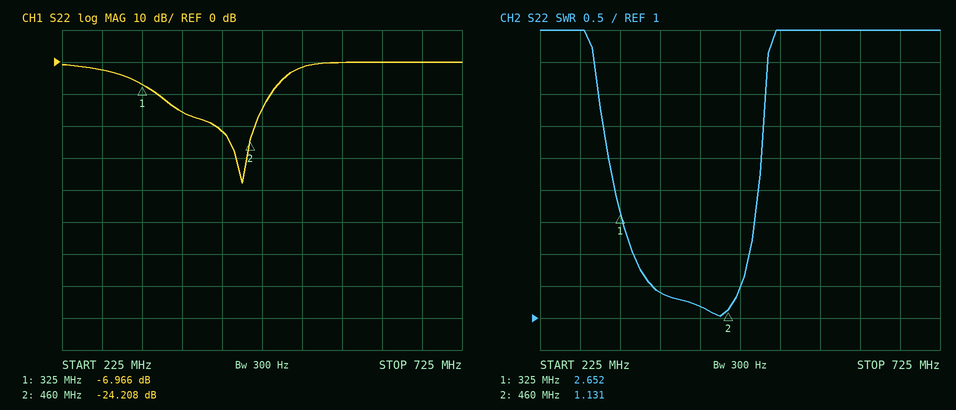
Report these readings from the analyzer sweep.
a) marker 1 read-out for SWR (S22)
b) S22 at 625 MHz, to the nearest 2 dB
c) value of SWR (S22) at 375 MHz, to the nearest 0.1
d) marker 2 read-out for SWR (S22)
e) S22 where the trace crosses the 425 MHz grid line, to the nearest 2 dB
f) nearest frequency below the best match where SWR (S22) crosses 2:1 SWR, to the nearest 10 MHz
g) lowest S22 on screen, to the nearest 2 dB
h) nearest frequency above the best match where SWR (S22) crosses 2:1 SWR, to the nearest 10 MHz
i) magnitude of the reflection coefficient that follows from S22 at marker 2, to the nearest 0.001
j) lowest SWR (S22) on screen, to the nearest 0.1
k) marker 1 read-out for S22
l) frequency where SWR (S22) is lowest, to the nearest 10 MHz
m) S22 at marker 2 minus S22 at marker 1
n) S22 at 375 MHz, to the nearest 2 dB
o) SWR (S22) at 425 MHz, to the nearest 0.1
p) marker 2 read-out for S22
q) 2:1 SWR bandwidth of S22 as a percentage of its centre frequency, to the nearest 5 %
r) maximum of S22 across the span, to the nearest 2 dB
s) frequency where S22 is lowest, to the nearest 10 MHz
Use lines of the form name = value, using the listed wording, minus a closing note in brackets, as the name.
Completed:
marker 1 read-out for SWR = 2.652
S22 at 625 MHz, to the nearest 2 dB = 0 dB
value of SWR (S22) at 375 MHz, to the nearest 0.1 = 1.4
marker 2 read-out for SWR = 1.131
S22 where the trace crosses the 425 MHz grid line, to the nearest 2 dB = -22 dB
nearest frequency below the best match where SWR (S22) crosses 2:1 SWR, to the nearest 10 MHz = 340 MHz
lowest S22 on screen, to the nearest 2 dB = -38 dB
nearest frequency above the best match where SWR (S22) crosses 2:1 SWR, to the nearest 10 MHz = 490 MHz
magnitude of the reflection coefficient that follows from S22 at marker 2, to the nearest 0.001 = 0.062
lowest SWR (S22) on screen, to the nearest 0.1 = 1.0
marker 1 read-out for S22 = -6.966 dB
frequency where SWR (S22) is lowest, to the nearest 10 MHz = 450 MHz
S22 at marker 2 minus S22 at marker 1 = -17.242 dB
S22 at 375 MHz, to the nearest 2 dB = -16 dB
SWR (S22) at 425 MHz, to the nearest 0.1 = 1.2
marker 2 read-out for S22 = -24.208 dB
2:1 SWR bandwidth of S22 as a percentage of its centre frequency, to the nearest 5 % = 35 %
maximum of S22 across the span, to the nearest 2 dB = 0 dB
frequency where S22 is lowest, to the nearest 10 MHz = 450 MHz
